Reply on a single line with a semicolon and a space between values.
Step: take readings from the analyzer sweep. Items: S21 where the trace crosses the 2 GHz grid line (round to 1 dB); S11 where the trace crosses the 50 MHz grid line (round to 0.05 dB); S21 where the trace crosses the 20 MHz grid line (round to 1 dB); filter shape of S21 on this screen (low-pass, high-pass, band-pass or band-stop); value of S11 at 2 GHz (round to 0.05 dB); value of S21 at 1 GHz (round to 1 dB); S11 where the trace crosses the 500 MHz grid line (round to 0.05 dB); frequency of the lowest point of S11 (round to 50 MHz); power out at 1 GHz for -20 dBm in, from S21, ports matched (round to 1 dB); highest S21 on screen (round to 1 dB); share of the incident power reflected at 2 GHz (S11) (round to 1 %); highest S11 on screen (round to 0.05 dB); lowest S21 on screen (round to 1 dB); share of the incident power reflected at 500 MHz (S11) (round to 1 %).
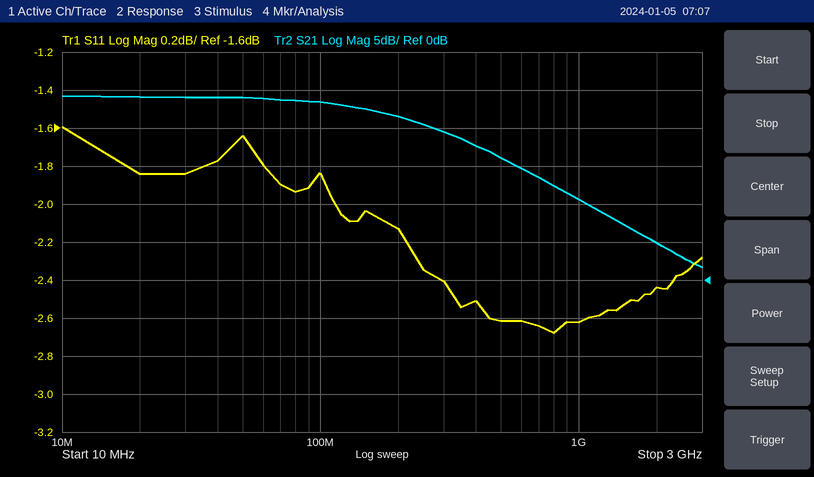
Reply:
5 dB; -1.65 dB; 24 dB; low-pass; -2.45 dB; 11 dB; -2.60 dB; 800 MHz; -9 dBm; 24 dB; 57 %; -1.60 dB; 2 dB; 55 %
